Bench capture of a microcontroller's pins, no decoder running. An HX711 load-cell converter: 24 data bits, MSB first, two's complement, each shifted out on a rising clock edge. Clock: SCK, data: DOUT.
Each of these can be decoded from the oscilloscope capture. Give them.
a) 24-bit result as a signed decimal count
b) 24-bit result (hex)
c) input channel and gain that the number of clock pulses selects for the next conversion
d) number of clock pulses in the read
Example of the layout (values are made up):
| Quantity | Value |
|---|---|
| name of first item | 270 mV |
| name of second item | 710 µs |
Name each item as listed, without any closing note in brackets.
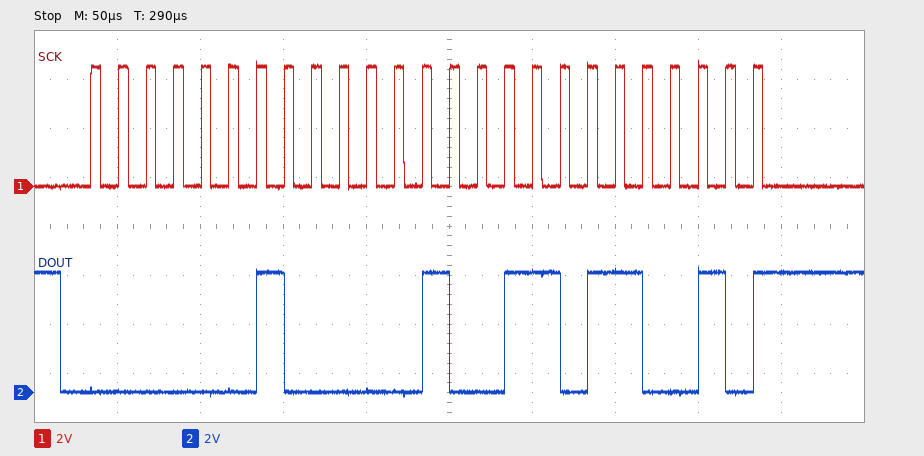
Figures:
| Quantity | Value |
|---|---|
| 24-bit result as a signed decimal count | 133554 |
| 24-bit result | 0x0209B2 |
| input channel and gain that the number of clock pulses selects for the next conversion | channel A, gain 128 |
| number of clock pulses in the read | 25 |
